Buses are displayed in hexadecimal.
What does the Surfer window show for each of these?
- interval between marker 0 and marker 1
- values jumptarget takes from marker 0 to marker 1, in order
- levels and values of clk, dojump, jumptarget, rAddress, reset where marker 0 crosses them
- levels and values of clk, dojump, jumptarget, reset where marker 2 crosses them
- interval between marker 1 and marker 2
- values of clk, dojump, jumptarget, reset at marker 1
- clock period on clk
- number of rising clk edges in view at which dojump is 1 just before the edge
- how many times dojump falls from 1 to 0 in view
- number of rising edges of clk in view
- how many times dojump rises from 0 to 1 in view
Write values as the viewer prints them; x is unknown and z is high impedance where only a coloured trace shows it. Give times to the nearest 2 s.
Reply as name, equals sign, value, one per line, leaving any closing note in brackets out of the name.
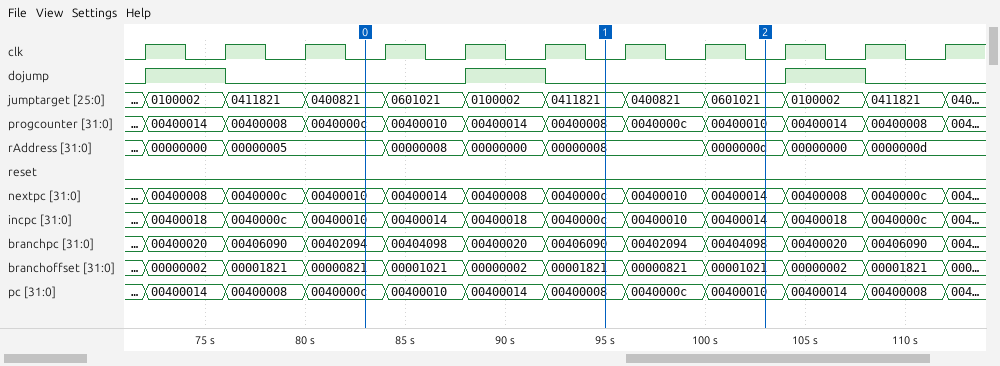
interval between marker 0 and marker 1 = 12 s
values jumptarget takes from marker 0 to marker 1, in order = 0400821, 0601021, 0100002, 0411821
levels and values of clk, dojump, jumptarget, rAddress, reset where marker 0 crosses them = clk=0, dojump=0, jumptarget=0400821, rAddress=00000005, reset=0
levels and values of clk, dojump, jumptarget, reset where marker 2 crosses them = clk=0, dojump=0, jumptarget=0601021, reset=0
interval between marker 1 and marker 2 = 8 s
values of clk, dojump, jumptarget, reset at marker 1 = clk=0, dojump=0, jumptarget=0411821, reset=0
clock period on clk = 4 s
number of rising clk edges in view at which dojump is 1 just before the edge = 3
how many times dojump falls from 1 to 0 in view = 3
number of rising edges of clk in view = 11
how many times dojump rises from 0 to 1 in view = 3
